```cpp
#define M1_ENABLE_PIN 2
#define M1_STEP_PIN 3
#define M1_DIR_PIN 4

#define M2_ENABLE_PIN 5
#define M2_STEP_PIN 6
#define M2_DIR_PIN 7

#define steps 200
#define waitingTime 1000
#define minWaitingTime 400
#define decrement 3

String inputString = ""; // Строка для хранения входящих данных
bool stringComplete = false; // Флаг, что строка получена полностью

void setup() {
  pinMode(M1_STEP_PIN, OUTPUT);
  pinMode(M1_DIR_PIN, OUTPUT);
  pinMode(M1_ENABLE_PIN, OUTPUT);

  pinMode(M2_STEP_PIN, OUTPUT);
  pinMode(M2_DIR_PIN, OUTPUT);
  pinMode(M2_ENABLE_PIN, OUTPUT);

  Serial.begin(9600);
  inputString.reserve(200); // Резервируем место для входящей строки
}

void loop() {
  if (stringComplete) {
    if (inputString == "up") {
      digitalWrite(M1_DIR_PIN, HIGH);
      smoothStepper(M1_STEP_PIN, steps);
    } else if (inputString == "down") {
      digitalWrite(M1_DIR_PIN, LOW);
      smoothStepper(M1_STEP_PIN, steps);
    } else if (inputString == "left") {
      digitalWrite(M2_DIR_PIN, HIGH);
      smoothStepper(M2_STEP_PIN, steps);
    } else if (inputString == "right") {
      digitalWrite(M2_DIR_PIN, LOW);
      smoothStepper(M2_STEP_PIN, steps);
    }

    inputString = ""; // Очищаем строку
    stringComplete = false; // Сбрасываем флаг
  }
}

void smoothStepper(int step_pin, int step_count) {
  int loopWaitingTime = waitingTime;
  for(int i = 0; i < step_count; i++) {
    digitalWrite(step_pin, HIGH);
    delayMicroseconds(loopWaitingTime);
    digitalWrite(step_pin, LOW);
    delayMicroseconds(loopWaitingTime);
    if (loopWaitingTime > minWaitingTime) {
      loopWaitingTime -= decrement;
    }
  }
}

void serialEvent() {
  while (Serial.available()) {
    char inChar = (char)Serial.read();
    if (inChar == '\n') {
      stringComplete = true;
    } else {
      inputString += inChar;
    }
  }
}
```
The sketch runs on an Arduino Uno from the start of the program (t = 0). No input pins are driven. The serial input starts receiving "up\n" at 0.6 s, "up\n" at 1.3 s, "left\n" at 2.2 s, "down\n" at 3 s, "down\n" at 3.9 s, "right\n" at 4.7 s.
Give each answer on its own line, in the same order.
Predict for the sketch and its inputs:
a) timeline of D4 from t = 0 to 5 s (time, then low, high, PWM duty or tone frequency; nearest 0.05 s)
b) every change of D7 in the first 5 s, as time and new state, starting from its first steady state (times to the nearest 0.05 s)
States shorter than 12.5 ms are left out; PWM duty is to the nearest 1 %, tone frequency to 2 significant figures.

0 s low; 0.6 s high; 3 s low
0 s low; 2.2 s high; 4.7 s low
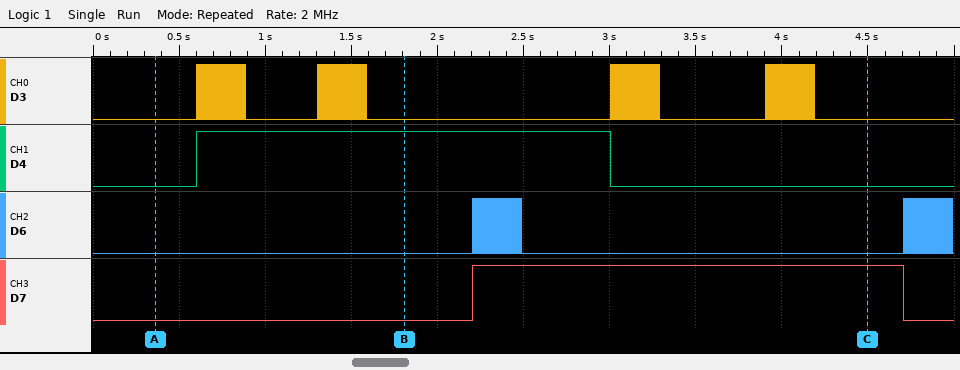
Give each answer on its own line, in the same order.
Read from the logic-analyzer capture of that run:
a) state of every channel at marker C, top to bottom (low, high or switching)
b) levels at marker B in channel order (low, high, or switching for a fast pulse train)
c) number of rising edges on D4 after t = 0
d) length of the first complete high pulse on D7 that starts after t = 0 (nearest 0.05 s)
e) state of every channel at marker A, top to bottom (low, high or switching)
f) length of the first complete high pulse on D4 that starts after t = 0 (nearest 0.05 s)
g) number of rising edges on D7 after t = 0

D3 low, D4 low, D6 low, D7 high
D3 low, D4 high, D6 low, D7 low
1
2.50 s
D3 low, D4 low, D6 low, D7 low
2.40 s
1
